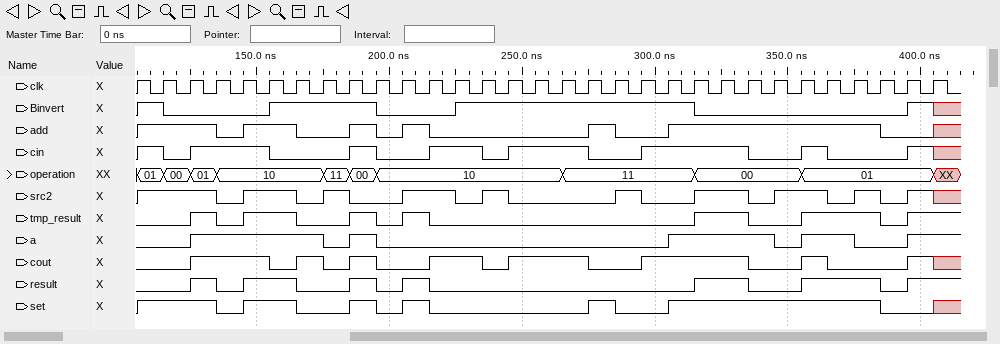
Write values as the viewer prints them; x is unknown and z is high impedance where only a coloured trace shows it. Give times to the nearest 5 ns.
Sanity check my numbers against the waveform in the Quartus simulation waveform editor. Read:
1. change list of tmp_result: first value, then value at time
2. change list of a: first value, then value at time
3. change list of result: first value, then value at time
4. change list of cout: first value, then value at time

0, 1 at 125 ns, 0 at 135 ns, 1 at 145 ns, 0 at 165 ns, 1 at 185 ns, 0 at 195 ns, 1 at 205 ns, 0 at 215 ns, 1 at 315 ns, 0 at 335 ns, 1 at 355 ns, 0 at 385 ns, 1 at 395 ns
0, 1 at 125 ns, 0 at 175 ns, 1 at 185 ns, 0 at 195 ns, 1 at 305 ns, 0 at 345 ns, 1 at 355 ns, 0 at 375 ns, 1 at 395 ns
0, 1 at 125 ns, 0 at 135 ns, 1 at 145 ns, 0 at 165 ns, 1 at 185 ns, 0 at 195 ns, 1 at 205 ns, 0 at 215 ns, 1 at 315 ns, 0 at 335 ns, 1 at 355 ns, 0 at 385 ns, 1 at 395 ns
0, 1 at 125 ns, 0 at 155 ns, 1 at 165 ns, 0 at 175 ns, 1 at 185 ns, 0 at 195 ns, 1 at 215 ns, 0 at 235 ns, 1 at 245 ns, 0 at 275 ns, 1 at 295 ns, 0 at 335 ns, 1 at 355 ns, 0 at 365 ns, 1 at 395 ns, x at 405 ns
